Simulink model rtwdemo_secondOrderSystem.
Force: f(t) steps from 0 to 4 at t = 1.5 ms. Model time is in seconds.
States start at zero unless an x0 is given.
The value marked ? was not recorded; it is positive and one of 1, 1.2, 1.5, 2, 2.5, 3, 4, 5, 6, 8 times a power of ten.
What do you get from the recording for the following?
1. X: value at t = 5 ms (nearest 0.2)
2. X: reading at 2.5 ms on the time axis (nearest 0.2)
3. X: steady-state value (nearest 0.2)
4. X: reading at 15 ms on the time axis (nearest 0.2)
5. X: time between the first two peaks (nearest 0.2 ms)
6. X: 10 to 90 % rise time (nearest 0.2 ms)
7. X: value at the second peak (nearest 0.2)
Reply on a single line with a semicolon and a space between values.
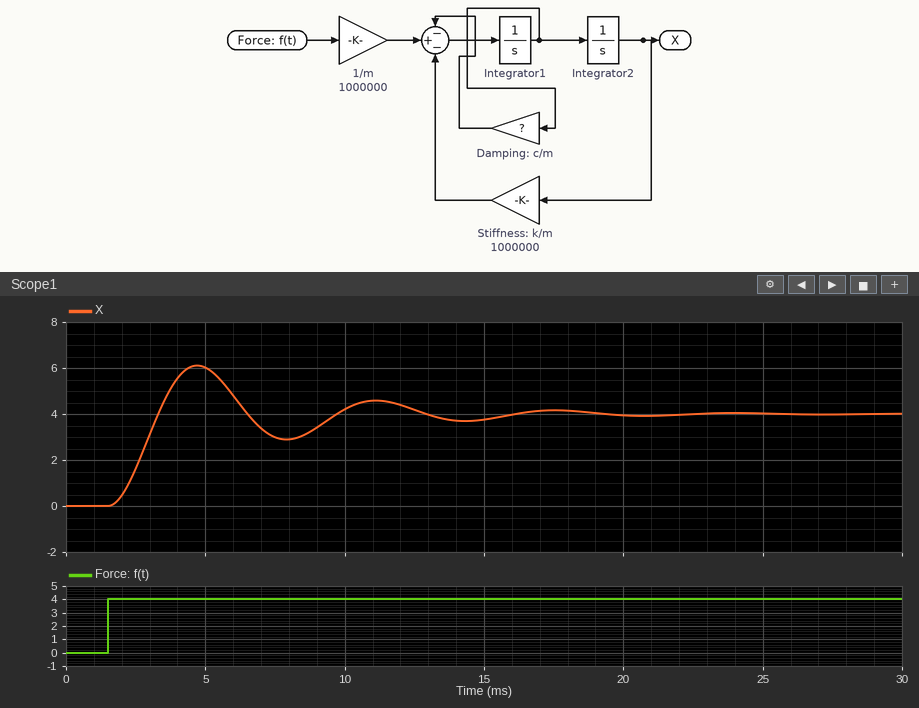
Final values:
6.0; 1.6; 4.0; 3.8; 6.4 ms; 1.2 ms; 4.6
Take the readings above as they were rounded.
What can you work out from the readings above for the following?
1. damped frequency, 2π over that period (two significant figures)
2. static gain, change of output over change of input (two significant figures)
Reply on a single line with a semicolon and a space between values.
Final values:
0.98 rad/ms; 1.0
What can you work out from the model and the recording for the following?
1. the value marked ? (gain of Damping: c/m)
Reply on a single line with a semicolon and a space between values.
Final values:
400
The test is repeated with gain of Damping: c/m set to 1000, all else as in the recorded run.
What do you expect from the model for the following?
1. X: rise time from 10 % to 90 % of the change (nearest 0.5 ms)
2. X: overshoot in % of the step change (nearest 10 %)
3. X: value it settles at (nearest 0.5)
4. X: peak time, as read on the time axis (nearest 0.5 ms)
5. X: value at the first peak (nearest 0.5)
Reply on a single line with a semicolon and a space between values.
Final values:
1.5 ms; 20 %; 4.0; 5.0 ms; 4.5
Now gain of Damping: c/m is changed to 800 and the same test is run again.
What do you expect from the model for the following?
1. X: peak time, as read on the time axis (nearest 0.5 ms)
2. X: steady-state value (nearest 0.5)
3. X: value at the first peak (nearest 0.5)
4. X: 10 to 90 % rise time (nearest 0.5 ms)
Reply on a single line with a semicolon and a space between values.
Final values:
5.0 ms; 4.0; 5.0; 1.5 ms
